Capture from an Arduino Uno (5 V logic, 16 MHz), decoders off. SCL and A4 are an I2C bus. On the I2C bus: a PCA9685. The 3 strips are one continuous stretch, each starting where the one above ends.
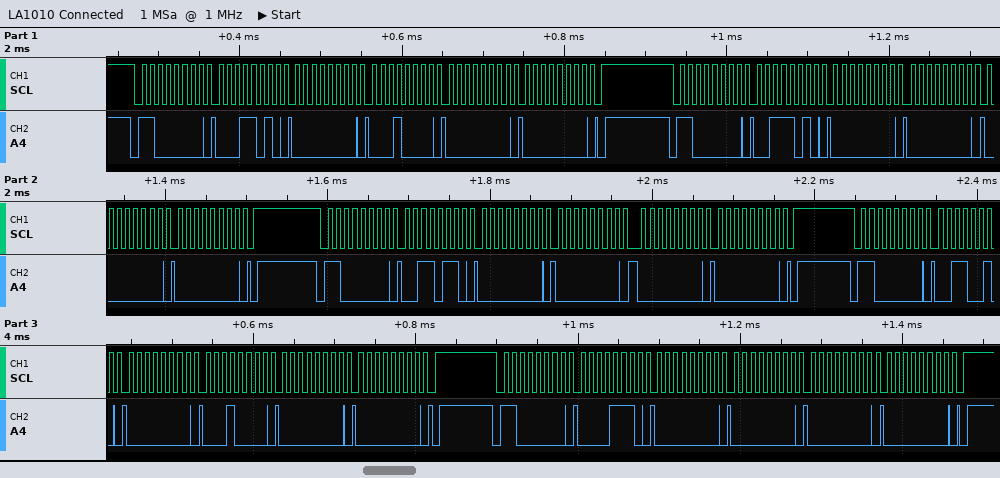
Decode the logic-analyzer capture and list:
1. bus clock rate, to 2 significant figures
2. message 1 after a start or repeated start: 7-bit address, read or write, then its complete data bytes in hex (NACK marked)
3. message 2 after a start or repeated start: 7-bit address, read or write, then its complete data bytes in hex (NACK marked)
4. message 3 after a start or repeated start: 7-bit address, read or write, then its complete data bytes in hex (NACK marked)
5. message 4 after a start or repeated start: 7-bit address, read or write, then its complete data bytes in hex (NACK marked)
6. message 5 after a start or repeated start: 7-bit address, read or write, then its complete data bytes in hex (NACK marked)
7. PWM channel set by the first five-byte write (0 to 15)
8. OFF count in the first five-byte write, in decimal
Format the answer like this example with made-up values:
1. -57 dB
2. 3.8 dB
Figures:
1. 100 kHz
2. 0x60 write: 1A 00 10 00 00
3. 0x60 write: 3A 00 00 00 00
4. 0x60 write: 36 00 00 00 00
5. 0x60 write: 32 00 10 00 00
6. 0x60 write: 0E 00 00 00 00
7. 5
8. 0
